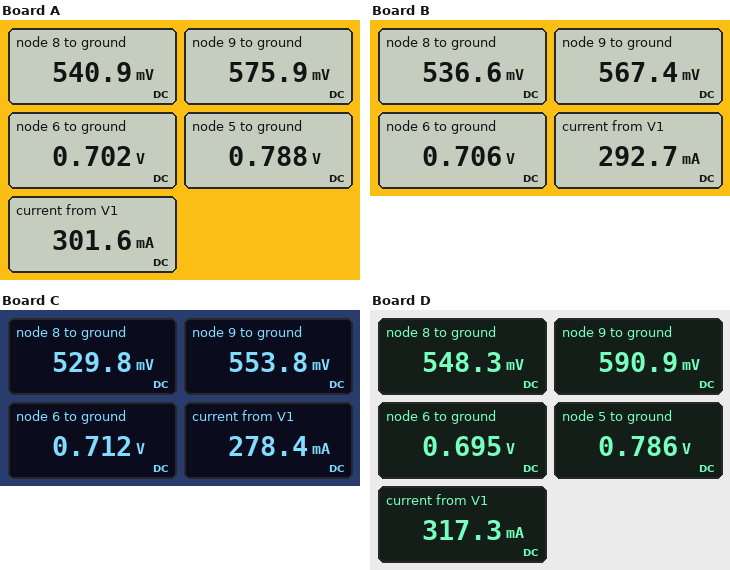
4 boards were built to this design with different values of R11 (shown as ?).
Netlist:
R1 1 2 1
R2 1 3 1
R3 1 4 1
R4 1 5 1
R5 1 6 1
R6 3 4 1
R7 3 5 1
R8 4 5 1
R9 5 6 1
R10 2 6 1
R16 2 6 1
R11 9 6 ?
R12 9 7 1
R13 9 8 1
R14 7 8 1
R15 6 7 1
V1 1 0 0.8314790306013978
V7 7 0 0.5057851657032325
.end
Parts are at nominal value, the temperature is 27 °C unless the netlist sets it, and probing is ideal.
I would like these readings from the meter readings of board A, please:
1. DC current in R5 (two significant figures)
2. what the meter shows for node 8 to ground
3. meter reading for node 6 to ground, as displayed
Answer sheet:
130 mA
540.9 mV
0.702 V
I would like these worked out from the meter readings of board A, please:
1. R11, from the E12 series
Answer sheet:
1.2 Ω
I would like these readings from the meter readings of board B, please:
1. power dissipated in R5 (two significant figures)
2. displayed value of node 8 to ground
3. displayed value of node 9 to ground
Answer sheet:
16 mW
536.6 mV
567.4 mV
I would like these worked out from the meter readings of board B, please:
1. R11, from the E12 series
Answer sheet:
1.5 Ω
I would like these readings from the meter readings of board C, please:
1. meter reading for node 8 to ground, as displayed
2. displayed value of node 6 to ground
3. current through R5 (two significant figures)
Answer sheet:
529.8 mV
0.712 V
120 mA
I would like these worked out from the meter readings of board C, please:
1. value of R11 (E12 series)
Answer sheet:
2.2 Ω
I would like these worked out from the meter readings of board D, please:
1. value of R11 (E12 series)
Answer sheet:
0.82 Ω
